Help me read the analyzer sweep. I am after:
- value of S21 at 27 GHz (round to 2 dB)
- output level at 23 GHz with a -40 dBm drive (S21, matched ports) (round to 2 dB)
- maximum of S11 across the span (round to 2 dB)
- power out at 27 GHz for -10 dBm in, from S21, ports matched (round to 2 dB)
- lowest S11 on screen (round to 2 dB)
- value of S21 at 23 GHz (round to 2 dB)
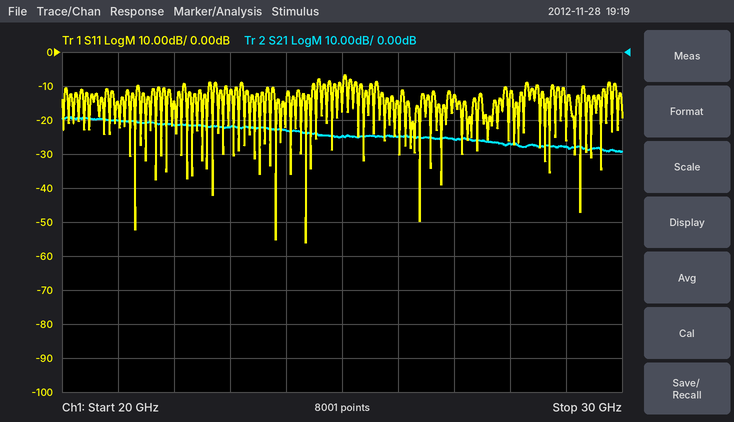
-26 dB
-62 dBm
-6 dB
-36 dBm
-56 dB
-22 dB
